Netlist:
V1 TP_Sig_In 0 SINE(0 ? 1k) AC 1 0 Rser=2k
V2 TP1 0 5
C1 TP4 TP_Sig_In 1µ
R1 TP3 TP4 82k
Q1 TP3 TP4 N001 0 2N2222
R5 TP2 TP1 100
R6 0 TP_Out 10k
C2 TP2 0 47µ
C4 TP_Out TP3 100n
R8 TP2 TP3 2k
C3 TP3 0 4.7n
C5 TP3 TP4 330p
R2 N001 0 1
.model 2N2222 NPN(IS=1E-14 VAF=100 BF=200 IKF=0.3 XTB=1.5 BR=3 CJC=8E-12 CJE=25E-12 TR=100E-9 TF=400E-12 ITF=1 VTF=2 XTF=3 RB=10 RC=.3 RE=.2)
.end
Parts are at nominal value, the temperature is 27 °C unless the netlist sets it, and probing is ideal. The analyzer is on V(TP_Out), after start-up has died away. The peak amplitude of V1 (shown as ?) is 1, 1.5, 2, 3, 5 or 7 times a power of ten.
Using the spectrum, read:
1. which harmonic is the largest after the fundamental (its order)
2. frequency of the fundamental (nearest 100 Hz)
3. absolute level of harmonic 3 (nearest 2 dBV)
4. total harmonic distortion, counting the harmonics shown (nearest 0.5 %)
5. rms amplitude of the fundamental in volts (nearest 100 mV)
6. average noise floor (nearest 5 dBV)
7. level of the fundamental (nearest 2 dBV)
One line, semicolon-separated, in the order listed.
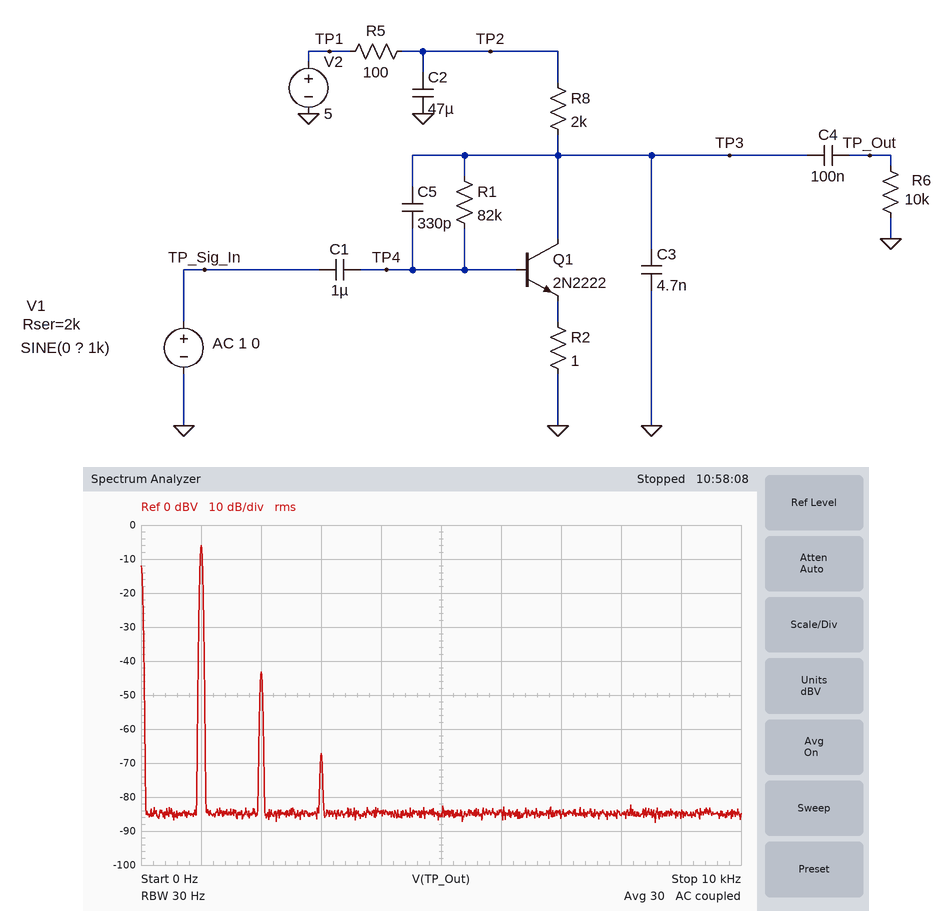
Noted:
2; 1.0 kHz; -68 dBV; 1.5 %; 500 mV; -85 dBV; -6 dBV
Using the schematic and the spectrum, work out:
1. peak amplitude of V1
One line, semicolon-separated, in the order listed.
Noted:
30 mV
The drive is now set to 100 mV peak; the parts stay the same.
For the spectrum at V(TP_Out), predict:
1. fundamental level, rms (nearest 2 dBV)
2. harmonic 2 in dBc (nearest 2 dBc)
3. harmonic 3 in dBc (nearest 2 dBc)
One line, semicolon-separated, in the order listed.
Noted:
2 dBV; -22 dBc; -20 dBc
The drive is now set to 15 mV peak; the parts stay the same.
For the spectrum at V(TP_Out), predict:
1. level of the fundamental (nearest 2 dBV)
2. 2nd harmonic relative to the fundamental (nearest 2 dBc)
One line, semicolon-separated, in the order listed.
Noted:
-12 dBV; -44 dBc
